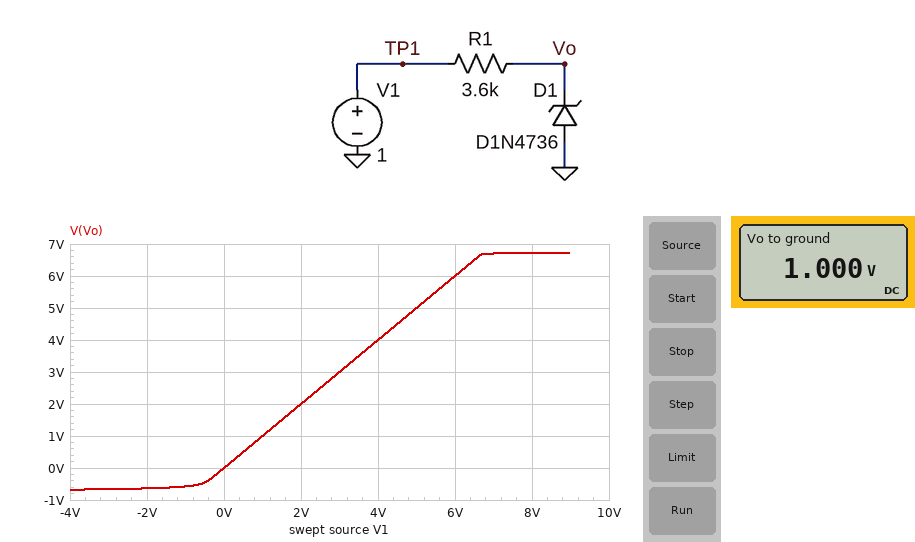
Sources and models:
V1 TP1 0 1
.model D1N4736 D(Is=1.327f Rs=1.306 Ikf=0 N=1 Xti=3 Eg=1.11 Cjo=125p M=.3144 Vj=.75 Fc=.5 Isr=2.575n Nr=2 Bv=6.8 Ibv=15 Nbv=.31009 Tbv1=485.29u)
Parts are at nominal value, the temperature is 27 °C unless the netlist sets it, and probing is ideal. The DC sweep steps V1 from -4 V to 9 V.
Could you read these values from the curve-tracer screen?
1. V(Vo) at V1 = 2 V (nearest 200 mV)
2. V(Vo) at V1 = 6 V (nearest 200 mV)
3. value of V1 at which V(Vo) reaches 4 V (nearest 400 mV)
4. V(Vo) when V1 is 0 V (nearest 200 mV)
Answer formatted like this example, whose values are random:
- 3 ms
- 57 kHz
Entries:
- 2.0 V
- 6.0 V
- 4.0 V
- 0 V
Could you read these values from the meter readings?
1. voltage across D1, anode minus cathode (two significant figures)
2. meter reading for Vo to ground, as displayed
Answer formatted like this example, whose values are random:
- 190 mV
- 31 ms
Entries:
- -1.0 V
- 1.000 V
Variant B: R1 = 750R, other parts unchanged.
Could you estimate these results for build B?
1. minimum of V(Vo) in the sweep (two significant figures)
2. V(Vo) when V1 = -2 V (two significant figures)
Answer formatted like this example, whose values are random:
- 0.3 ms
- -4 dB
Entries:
- -740 mV
- -700 mV
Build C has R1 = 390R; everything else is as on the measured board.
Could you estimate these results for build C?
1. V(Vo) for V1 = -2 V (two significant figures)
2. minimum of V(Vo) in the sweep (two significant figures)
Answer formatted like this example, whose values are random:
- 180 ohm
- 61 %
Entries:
- -730 mV
- -760 mV
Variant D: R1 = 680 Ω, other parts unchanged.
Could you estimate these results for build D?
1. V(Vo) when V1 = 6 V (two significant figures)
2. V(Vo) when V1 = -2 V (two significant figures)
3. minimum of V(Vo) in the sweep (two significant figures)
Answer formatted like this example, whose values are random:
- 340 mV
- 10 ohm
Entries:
- 6.0 V
- -710 mV
- -740 mV
